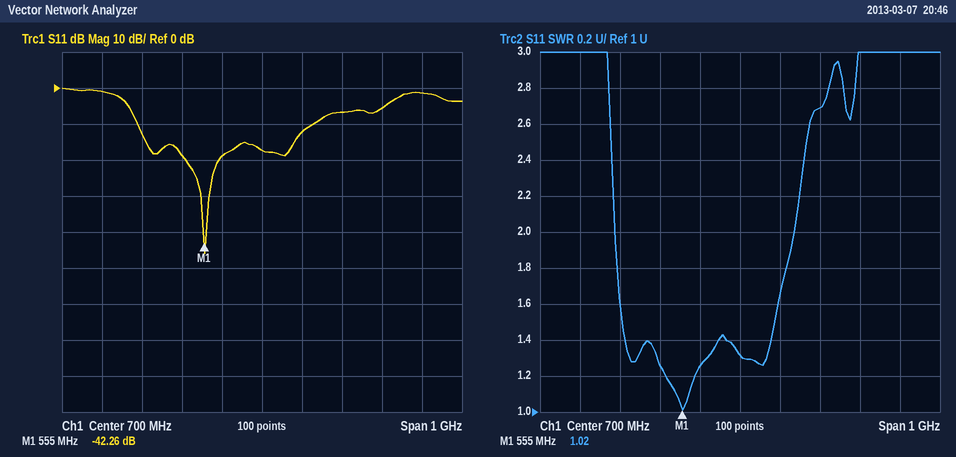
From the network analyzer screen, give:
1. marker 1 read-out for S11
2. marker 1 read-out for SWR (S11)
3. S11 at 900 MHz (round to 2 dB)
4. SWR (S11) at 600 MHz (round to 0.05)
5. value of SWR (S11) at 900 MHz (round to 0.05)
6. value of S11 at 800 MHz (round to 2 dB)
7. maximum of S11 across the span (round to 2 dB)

-42.26 dB
1.02
-6 dB
1.25
2.70
-12 dB
0 dB
